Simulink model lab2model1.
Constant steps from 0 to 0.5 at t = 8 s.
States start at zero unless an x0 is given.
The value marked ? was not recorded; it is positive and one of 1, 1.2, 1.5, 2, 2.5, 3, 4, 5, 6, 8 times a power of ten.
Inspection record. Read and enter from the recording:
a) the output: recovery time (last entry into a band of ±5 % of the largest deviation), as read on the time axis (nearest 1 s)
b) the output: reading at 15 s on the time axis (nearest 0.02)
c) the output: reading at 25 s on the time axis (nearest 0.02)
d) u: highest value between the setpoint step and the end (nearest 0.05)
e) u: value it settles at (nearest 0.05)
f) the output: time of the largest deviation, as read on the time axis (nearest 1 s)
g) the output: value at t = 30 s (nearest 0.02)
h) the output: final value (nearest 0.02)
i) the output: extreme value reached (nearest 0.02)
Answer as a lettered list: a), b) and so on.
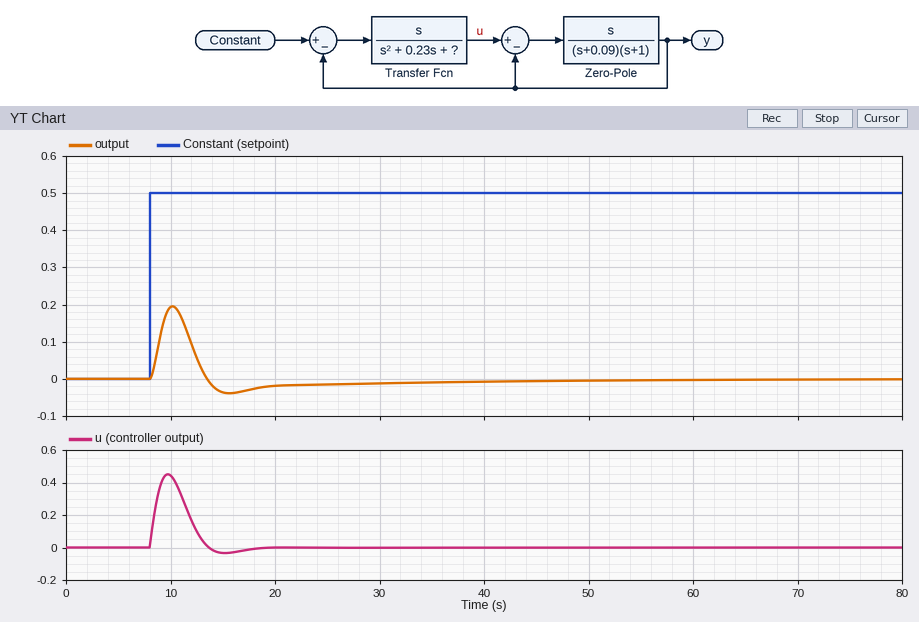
a) 35 s
b) -0.04
c) -0.02
d) 0.45
e) 0.00
f) 10 s
g) -0.02
h) 0.00
i) 0.20
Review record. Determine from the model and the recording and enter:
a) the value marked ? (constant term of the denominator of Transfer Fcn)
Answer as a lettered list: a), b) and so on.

a) 0.4
